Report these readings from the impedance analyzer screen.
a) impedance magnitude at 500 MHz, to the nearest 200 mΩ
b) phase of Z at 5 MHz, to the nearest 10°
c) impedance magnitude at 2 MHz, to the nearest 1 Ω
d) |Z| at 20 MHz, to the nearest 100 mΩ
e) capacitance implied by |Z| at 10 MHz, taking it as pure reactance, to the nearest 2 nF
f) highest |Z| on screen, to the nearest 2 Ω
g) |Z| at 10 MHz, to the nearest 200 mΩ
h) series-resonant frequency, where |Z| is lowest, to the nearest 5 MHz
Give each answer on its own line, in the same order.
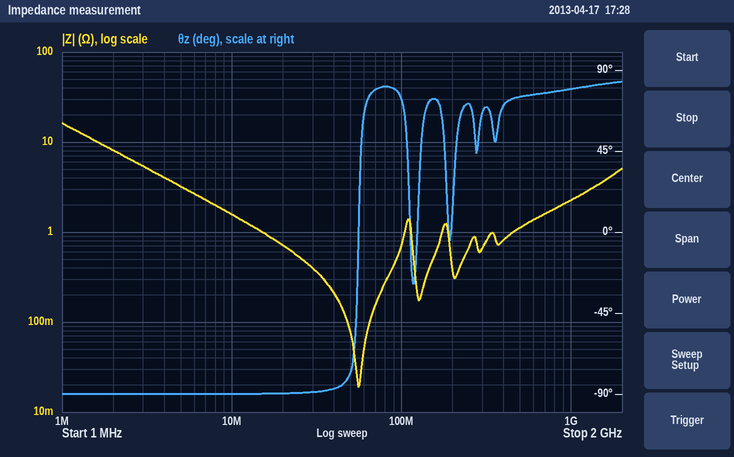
1.2 Ω
-90°
8 Ω
700 mΩ
10 nF
16 Ω
1.6 Ω
55 MHz
